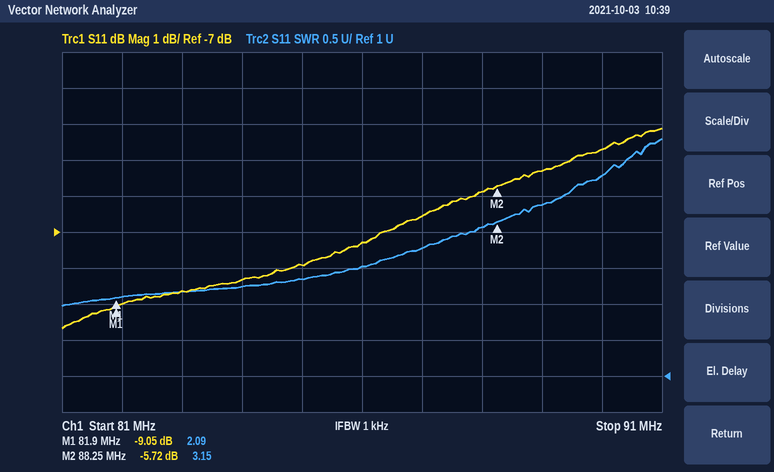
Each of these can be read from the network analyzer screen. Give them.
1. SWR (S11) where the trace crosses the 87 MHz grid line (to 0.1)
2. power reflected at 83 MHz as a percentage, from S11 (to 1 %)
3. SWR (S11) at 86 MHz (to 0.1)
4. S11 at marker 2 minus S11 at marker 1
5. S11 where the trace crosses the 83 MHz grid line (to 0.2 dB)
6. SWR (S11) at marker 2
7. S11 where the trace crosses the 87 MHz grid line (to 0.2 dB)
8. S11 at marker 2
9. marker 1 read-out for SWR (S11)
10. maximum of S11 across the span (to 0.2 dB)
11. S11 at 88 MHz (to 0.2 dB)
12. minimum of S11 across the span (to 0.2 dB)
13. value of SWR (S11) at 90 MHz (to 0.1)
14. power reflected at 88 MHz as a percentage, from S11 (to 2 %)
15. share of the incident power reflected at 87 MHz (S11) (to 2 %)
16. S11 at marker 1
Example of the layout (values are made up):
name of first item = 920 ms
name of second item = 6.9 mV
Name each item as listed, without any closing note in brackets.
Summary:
SWR (S11) where the trace crosses the 87 MHz grid line = 2.8
power reflected at 83 MHz as a percentage, from S11 = 14 %
SWR (S11) at 86 MHz = 2.5
S11 at marker 2 minus S11 at marker 1 = 3.33 dB
S11 where the trace crosses the 83 MHz grid line = -8.6 dB
SWR (S11) at marker 2 = 3.15
S11 where the trace crosses the 87 MHz grid line = -6.6 dB
S11 at marker 2 = -5.72 dB
marker 1 read-out for SWR = 2.09
maximum of S11 across the span = -4.2 dB
S11 at 88 MHz = -5.8 dB
minimum of S11 across the span = -9.6 dB
value of SWR (S11) at 90 MHz = 3.8
power reflected at 88 MHz as a percentage, from S11 = 26 %
share of the incident power reflected at 87 MHz (S11) = 22 %
S11 at marker 1 = -9.05 dB
